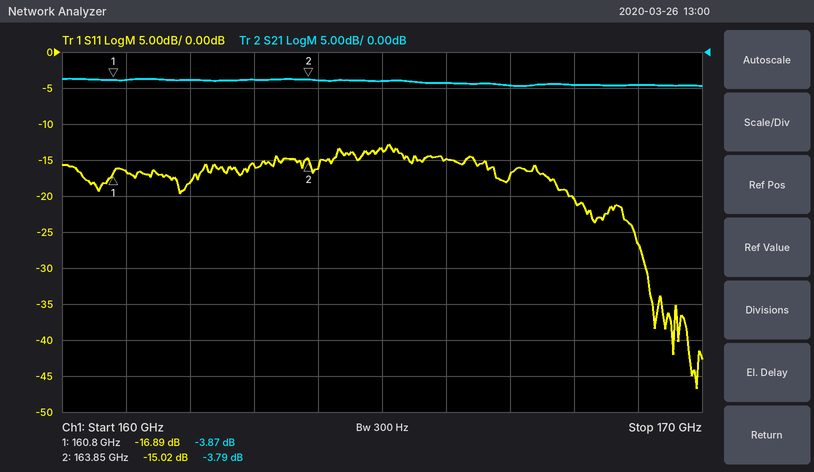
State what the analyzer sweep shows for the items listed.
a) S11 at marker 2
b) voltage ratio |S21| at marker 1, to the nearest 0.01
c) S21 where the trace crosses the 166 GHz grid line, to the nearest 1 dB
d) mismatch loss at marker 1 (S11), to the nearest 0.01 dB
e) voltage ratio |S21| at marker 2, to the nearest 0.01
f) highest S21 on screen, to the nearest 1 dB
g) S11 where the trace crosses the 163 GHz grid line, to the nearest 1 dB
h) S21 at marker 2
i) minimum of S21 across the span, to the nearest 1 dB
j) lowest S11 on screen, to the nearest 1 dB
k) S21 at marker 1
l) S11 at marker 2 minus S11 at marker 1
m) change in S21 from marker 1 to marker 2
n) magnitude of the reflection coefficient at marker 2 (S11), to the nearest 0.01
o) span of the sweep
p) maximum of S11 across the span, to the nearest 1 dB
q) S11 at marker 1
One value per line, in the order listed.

-15.02 dB
0.64
-4 dB
0.09 dB
0.65
-4 dB
-16 dB
-3.79 dB
-5 dB
-47 dB
-3.87 dB
1.87 dB
0.08 dB
0.18
10 GHz
-13 dB
-16.89 dB
